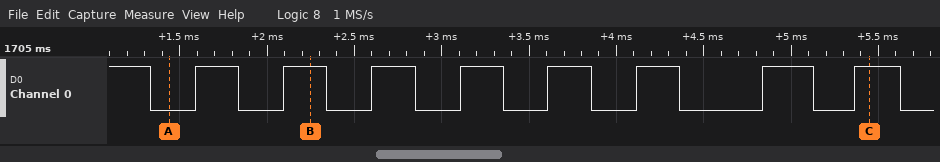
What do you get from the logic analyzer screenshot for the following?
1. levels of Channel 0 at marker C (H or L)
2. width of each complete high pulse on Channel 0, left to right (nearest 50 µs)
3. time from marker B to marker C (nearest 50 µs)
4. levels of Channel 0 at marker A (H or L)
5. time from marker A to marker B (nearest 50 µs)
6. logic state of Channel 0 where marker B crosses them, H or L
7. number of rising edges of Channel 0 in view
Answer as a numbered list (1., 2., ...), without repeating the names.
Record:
1. Channel 0=H
2. 250 µs, 250 µs, 250 µs, 250 µs, 250 µs, 250 µs, 300 µs, 250 µs
3. 3200 µs
4. Channel 0=L
5. 800 µs
6. Channel 0=H
7. 8
